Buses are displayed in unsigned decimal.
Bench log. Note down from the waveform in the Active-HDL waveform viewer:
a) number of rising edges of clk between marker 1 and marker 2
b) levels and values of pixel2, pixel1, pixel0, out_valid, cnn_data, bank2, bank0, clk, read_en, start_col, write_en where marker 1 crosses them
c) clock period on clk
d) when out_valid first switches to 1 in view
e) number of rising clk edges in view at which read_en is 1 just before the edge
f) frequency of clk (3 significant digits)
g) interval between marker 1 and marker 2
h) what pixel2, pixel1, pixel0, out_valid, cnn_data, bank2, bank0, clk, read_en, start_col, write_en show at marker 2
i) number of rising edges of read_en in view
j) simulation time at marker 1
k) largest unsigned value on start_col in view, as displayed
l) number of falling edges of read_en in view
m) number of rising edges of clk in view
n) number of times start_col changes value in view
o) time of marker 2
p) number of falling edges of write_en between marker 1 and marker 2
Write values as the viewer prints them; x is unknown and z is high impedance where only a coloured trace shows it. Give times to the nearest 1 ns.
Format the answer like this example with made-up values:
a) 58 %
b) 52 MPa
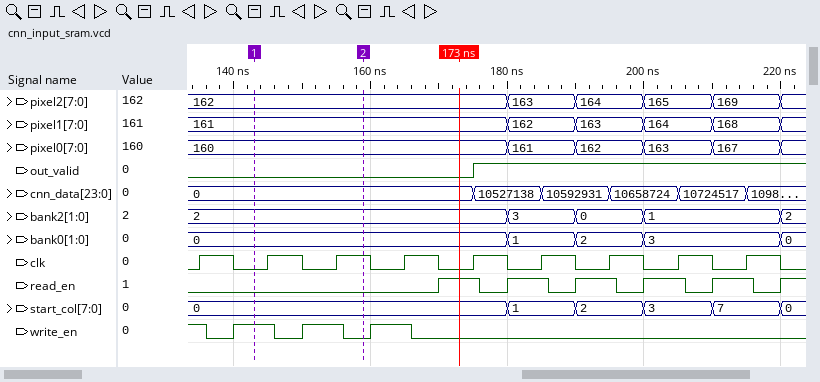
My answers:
a) 2
b) pixel2=162, pixel1=161, pixel0=160, out_valid=0, cnn_data=0, bank2=2, bank0=0, clk=0, read_en=0, start_col=0, write_en=1
c) 10 ns
d) 175 ns
e) 5
f) 100 MHz
g) 16 ns
h) pixel2=162, pixel1=161, pixel0=160, out_valid=0, cnn_data=0, bank2=2, bank0=0, clk=1, read_en=0, start_col=0, write_en=0
i) 6
j) 143 ns
k) 7
l) 5
m) 9
n) 5
o) 159 ns
p) 2
